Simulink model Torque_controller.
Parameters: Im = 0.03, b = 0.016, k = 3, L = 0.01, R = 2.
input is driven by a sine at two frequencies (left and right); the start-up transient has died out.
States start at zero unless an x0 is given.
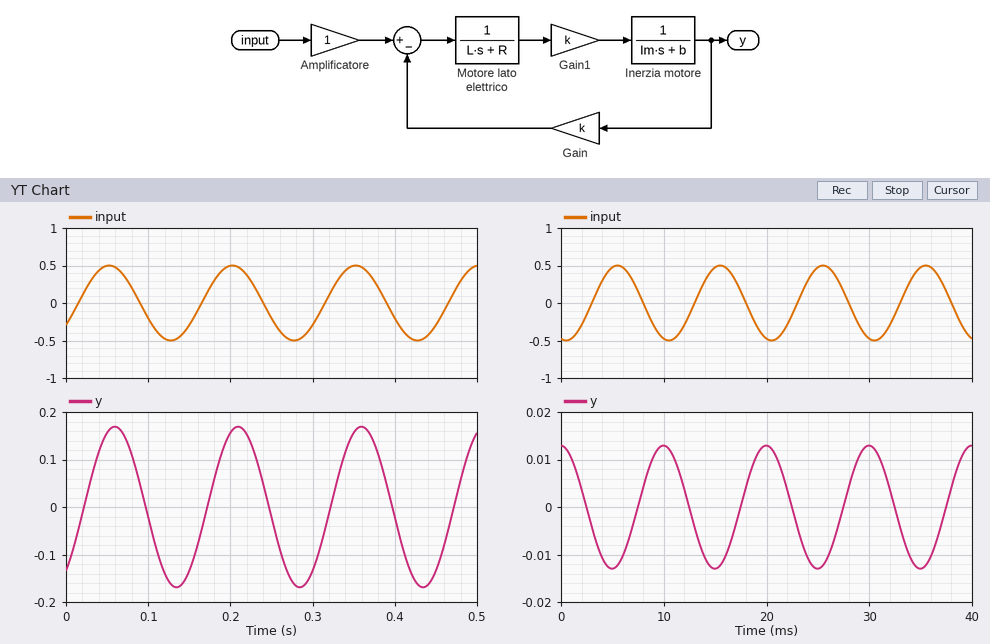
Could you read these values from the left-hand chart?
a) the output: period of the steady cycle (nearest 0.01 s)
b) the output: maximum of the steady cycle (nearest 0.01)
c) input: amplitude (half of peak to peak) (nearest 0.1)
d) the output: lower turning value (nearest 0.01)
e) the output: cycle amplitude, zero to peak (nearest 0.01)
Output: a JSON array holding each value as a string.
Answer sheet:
["0.15 s", "0.17", "0.5", "-0.17", "0.17"]
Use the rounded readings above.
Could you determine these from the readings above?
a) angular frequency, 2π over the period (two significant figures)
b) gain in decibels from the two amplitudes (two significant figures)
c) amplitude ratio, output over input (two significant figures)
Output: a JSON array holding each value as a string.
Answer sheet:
["42 rad/s", "-9.4 dB", "0.34"]
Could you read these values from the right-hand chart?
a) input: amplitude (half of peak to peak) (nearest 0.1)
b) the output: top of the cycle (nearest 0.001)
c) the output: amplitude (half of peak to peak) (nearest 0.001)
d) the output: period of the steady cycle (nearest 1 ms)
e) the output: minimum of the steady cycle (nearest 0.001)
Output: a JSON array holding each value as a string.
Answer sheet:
["0.5", "0.013", "0.013", "10 ms", "-0.013"]
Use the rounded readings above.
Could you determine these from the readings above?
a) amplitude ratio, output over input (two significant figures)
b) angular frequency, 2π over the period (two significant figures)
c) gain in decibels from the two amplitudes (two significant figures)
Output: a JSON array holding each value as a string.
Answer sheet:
["0.026", "0.63 rad/ms", "-32 dB"]
